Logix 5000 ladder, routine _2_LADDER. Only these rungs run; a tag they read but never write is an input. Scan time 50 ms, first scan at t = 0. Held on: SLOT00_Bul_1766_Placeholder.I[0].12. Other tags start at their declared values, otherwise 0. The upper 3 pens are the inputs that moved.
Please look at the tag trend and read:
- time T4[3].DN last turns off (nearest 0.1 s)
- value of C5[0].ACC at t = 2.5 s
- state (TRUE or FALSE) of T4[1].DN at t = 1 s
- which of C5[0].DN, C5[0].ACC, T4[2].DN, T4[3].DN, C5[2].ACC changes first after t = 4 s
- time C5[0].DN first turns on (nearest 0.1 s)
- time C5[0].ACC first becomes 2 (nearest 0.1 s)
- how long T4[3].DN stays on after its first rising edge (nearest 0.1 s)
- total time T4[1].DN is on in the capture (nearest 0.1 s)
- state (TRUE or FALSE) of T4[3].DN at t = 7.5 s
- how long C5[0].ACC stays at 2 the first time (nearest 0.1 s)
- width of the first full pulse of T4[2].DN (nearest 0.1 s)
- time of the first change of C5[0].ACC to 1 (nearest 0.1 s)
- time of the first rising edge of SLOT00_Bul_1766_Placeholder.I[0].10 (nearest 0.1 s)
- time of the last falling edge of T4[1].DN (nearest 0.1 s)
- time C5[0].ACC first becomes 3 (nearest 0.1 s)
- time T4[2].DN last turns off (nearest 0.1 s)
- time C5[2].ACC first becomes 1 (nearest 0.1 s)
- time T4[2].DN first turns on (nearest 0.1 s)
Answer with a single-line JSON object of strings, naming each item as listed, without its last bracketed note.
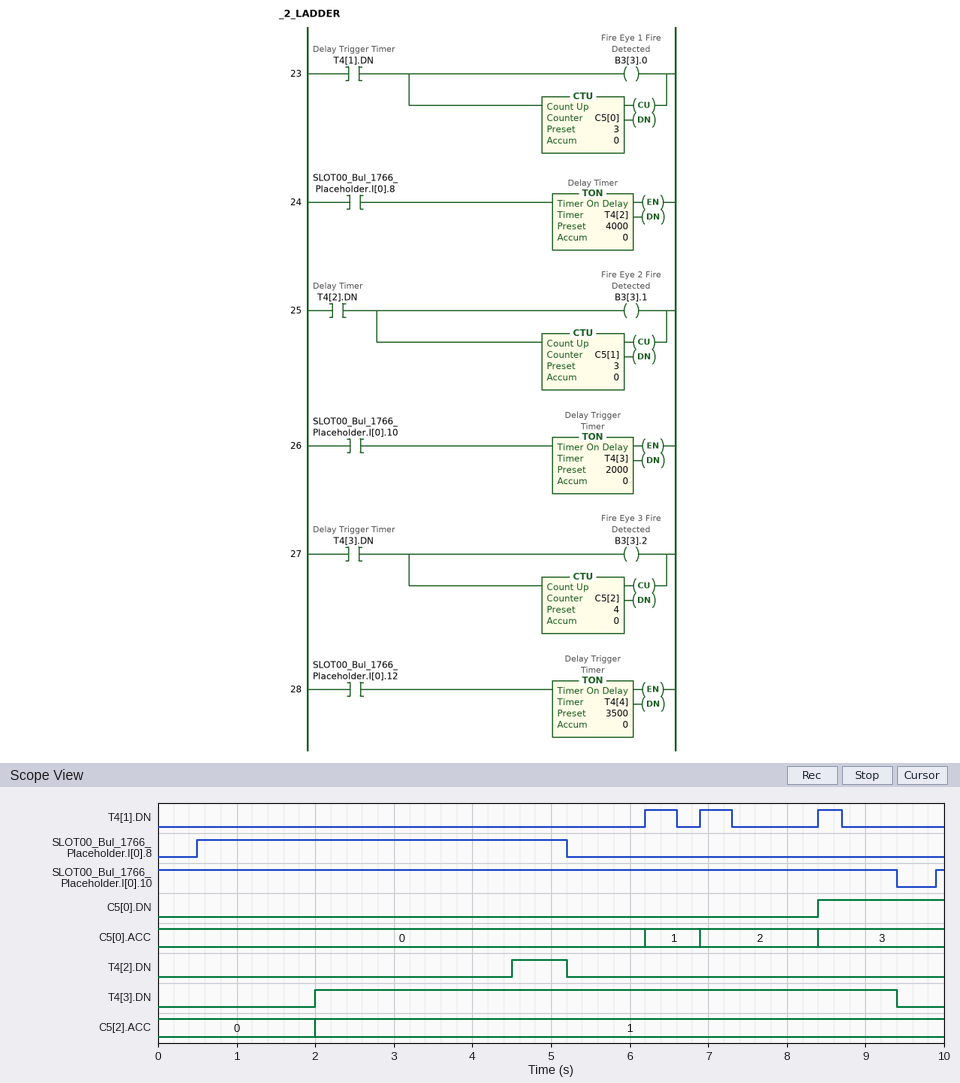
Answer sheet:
{"time T4[3].DN last turns off": "9.4 s", "value of C5[0].ACC at t = 2.5 s": "0", "state (TRUE or FALSE) of T4[1].DN at t = 1 s": "FALSE", "which of C5[0].DN, C5[0].ACC, T4[2].DN, T4[3].DN, C5[2].ACC changes first after t = 4 s": "T4[2].DN", "time C5[0].DN first turns on": "8.4 s", "time C5[0].ACC first becomes 2": "6.9 s", "how long T4[3].DN stays on after its first rising edge": "7.4 s", "total time T4[1].DN is on in the capture": "1.1 s", "state (TRUE or FALSE) of T4[3].DN at t = 7.5 s": "TRUE", "how long C5[0].ACC stays at 2 the first time": "1.5 s", "width of the first full pulse of T4[2].DN": "0.7 s", "time of the first change of C5[0].ACC to 1": "6.2 s", "time of the first rising edge of SLOT00_Bul_1766_Placeholder.I[0].10": "9.9 s", "time of the last falling edge of T4[1].DN": "8.7 s", "time C5[0].ACC first becomes 3": "8.4 s", "time T4[2].DN last turns off": "5.2 s", "time C5[2].ACC first becomes 1": "2.0 s", "time T4[2].DN first turns on": "4.5 s"}
